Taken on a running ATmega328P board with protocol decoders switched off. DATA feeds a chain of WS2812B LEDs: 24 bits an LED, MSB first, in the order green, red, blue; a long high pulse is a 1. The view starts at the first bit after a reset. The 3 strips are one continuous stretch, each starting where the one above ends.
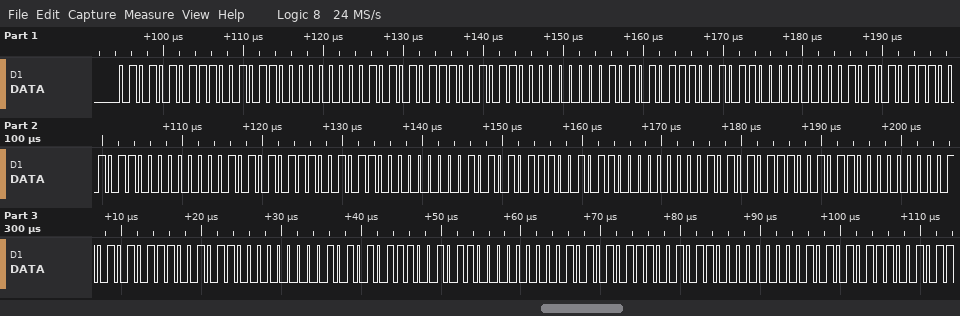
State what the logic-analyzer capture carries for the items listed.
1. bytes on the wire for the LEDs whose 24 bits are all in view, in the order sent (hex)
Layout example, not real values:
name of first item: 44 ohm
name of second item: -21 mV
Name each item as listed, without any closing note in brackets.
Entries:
bytes on the wire for the LEDs whose 24 bits are all in view, in the order sent: 55 CB 00 55 CB 00 55 CB 00 55 CB 00 55 CB 00 55 CB 00 55 CB 00 55 CB 00 55 CB 00 55 CB 00
